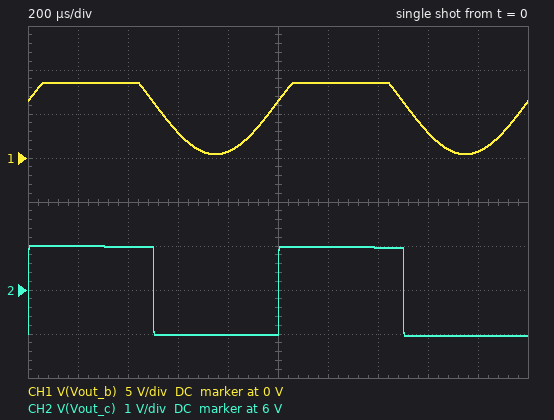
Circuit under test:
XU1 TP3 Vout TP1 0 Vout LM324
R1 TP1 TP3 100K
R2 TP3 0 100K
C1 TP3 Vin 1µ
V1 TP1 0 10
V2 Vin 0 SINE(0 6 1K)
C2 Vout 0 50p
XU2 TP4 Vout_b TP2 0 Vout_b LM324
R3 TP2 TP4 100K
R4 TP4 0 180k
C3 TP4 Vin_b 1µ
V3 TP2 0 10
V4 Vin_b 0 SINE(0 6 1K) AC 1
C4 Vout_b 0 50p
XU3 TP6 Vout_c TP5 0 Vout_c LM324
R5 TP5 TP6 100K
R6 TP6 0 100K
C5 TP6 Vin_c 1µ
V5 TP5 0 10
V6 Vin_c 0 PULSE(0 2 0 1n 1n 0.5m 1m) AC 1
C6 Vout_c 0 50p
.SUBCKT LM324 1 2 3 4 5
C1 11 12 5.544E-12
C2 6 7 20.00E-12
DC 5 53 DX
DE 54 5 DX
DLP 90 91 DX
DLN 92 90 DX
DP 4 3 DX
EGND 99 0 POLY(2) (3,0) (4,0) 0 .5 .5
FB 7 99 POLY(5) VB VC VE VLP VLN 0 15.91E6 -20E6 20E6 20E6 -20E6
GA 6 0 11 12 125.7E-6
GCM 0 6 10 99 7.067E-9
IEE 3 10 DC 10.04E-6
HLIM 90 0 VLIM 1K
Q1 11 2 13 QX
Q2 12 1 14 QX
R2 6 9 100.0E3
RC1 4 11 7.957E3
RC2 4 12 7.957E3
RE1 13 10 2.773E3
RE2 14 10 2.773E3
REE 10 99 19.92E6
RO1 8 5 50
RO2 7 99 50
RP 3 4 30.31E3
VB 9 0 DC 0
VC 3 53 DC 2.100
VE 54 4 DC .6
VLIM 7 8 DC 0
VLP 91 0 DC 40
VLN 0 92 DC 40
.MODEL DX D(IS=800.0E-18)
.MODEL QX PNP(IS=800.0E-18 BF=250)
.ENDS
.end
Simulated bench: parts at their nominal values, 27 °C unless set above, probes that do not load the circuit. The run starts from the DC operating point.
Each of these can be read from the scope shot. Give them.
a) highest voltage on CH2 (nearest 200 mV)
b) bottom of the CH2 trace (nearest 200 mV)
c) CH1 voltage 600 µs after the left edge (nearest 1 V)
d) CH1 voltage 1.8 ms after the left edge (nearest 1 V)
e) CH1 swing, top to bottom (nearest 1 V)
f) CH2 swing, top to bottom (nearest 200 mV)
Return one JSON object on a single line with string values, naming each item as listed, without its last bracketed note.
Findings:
{"highest voltage on CH2": "7.0 V", "bottom of the CH2 trace": "5.0 V", "CH1 voltage 600 µs after the left edge": "3 V", "CH1 voltage 1.8 ms after the left edge": "1 V", "CH1 swing, top to bottom": "8 V", "CH2 swing, top to bottom": "2.0 V"}
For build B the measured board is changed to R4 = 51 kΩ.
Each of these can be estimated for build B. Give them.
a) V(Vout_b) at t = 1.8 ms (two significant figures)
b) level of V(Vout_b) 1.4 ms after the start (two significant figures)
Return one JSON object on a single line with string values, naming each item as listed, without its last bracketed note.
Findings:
{"V(Vout_b) at t = 1.8 ms": "8.6 V", "level of V(Vout_b) 1.4 ms after the start": "6.9 V"}
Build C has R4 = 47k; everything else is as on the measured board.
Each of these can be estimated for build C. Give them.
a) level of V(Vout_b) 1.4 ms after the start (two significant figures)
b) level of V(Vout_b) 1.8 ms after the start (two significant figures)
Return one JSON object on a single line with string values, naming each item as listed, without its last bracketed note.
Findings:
{"level of V(Vout_b) 1.4 ms after the start": "6.7 V", "level of V(Vout_b) 1.8 ms after the start": "8.6 V"}
